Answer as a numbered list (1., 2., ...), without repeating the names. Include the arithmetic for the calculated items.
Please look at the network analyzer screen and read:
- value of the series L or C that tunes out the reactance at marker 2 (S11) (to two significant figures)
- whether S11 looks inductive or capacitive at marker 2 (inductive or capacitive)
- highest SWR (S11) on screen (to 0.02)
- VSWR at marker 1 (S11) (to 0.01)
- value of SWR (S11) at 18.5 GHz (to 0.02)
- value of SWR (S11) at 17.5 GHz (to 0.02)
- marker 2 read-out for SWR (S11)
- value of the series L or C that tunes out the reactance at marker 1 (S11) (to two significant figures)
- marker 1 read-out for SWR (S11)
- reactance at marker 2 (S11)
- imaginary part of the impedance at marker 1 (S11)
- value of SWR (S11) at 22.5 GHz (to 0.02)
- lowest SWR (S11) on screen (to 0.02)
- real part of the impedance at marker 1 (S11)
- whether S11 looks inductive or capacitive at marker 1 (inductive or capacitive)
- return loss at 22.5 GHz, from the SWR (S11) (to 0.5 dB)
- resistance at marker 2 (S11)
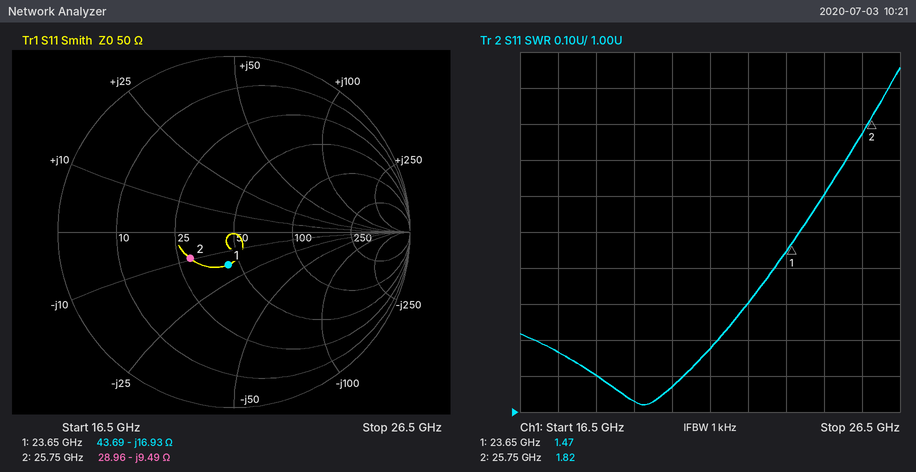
1. L = 9.49 Ω/(2π × 25.75 GHz) ≈ 59 pH
2. capacitive
3. 1.96
4. 1.47
5. 1.10
6. 1.16
7. 1.82
8. L = 16.93 Ω/(2π × 23.65 GHz) ≈ 114 pH, so 110 pH to two significant figures
9. 1.47
10. -9.49 Ω
11. -16.93 Ω
12. 1.30
13. 1.02
14. 43.69 Ω
15. capacitive
16. −20 log10((1.3 − 1)/(1.3 + 1)) ≈ 17.7 dB, so 17.5 dB to the nearest 0.5 dB
17. 28.96 Ω
